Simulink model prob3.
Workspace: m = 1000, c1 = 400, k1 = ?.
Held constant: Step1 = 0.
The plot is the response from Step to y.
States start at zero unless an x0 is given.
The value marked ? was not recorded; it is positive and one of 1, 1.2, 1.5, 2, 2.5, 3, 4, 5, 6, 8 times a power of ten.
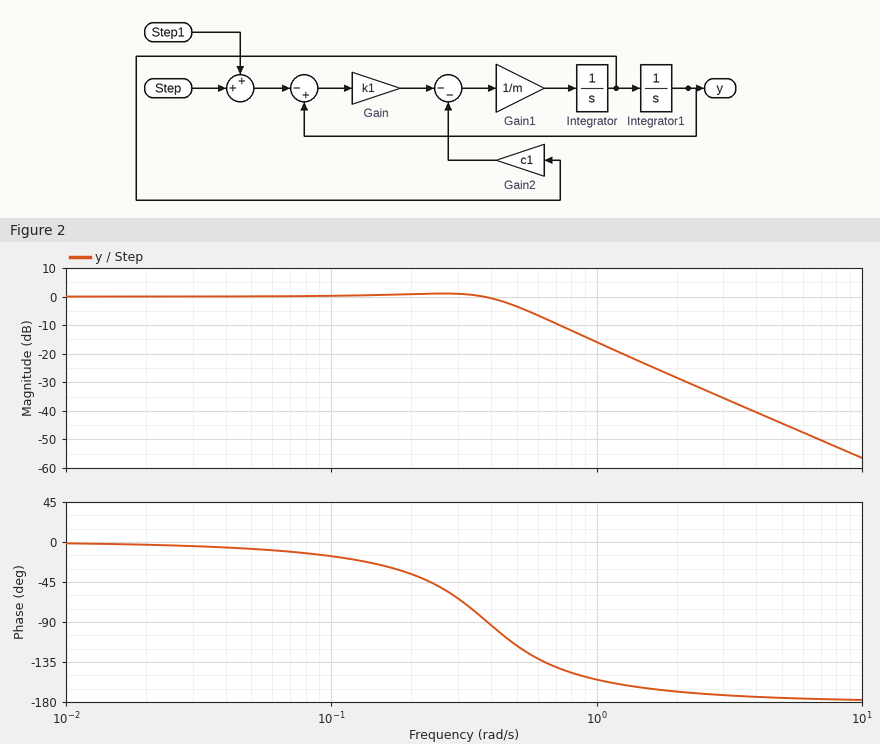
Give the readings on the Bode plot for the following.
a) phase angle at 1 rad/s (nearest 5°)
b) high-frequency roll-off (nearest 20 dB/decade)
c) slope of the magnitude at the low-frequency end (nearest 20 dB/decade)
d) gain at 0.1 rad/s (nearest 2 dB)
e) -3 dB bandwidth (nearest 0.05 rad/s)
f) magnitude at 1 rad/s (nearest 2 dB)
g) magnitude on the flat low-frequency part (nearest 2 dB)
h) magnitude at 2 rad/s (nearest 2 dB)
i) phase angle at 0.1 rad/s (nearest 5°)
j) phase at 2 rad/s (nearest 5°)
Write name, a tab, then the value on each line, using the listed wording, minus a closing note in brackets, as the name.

phase angle at 1 rad/s	-155°
high-frequency roll-off	-40 dB/decade
slope of the magnitude at the low-frequency end	0 dB/decade
gain at 0.1 rad/s	0 dB
-3 dB bandwidth	0.50 rad/s
magnitude at 1 rad/s	-16 dB
magnitude on the flat low-frequency part	0 dB
magnitude at 2 rad/s	-28 dB
phase angle at 0.1 rad/s	-15°
phase at 2 rad/s	-170°
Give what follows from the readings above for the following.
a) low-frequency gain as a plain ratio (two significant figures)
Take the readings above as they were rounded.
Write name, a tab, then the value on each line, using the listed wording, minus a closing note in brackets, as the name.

low-frequency gain as a plain ratio	1.0
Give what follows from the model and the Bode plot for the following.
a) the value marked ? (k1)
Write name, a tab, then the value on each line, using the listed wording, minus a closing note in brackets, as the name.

the value marked ?	150
